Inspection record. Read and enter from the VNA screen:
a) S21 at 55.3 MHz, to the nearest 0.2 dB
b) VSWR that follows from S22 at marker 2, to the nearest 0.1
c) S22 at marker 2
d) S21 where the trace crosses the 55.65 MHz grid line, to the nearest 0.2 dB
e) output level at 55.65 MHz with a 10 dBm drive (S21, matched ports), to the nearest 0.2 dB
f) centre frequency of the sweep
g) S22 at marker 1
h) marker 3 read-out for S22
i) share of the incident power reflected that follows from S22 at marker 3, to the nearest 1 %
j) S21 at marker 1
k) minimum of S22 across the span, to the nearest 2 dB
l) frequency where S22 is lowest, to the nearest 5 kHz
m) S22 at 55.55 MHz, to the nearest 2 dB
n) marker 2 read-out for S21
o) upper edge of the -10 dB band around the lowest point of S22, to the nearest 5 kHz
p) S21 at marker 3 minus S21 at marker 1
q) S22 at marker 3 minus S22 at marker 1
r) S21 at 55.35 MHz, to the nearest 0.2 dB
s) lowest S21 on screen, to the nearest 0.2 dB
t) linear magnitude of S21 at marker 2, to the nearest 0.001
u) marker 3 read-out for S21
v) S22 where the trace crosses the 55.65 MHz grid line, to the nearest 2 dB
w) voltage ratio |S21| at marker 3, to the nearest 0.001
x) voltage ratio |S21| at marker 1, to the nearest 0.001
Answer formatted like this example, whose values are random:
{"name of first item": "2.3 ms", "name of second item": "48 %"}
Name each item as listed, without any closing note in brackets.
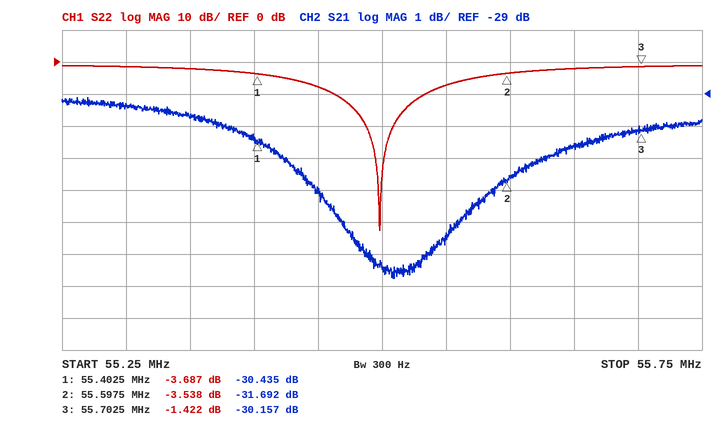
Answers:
{"S21 at 55.3 MHz, to the nearest 0.2 dB": "-29.4 dB", "VSWR that follows from S22 at marker 2, to the nearest 0.1": "5.0", "S22 at marker 2": "-3.538 dB", "S21 where the trace crosses the 55.65 MHz grid line, to the nearest 0.2 dB": "-30.6 dB", "output level at 55.65 MHz with a 10 dBm drive (S21, matched ports), to the nearest 0.2 dB": "-20.6 dBm", "centre frequency of the sweep": "55.5 MHz", "S22 at marker 1": "-3.687 dB", "marker 3 read-out for S22": "-1.422 dB", "share of the incident power reflected that follows from S22 at marker 3, to the nearest 1 %": "72 %", "S21 at marker 1": "-30.435 dB", "minimum of S22 across the span, to the nearest 2 dB": "-52 dB", "frequency where S22 is lowest, to the nearest 5 kHz": "55.500 MHz", "S22 at 55.55 MHz, to the nearest 2 dB": "-8 dB", "marker 2 read-out for S21": "-31.692 dB", "upper edge of the -10 dB band around the lowest point of S22, to the nearest 5 kHz": "55.535 MHz", "S21 at marker 3 minus S21 at marker 1": "0.278 dB", "S22 at marker 3 minus S22 at marker 1": "2.265 dB", "S21 at 55.35 MHz, to the nearest 0.2 dB": "-29.8 dB", "lowest S21 on screen, to the nearest 0.2 dB": "-34.8 dB", "linear magnitude of S21 at marker 2, to the nearest 0.001": "0.026", "marker 3 read-out for S21": "-30.157 dB", "S22 where the trace crosses the 55.65 MHz grid line, to the nearest 2 dB": "-2 dB", "voltage ratio |S21| at marker 3, to the nearest 0.001": "0.031", "voltage ratio |S21| at marker 1, to the nearest 0.001": "0.030"}
